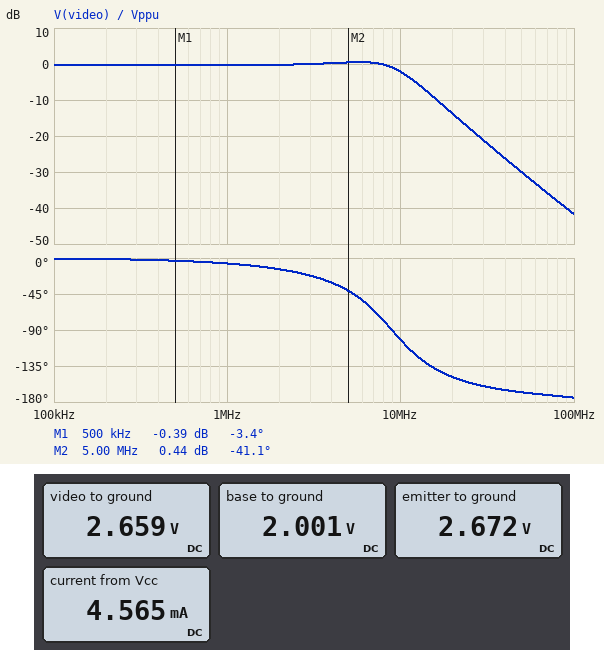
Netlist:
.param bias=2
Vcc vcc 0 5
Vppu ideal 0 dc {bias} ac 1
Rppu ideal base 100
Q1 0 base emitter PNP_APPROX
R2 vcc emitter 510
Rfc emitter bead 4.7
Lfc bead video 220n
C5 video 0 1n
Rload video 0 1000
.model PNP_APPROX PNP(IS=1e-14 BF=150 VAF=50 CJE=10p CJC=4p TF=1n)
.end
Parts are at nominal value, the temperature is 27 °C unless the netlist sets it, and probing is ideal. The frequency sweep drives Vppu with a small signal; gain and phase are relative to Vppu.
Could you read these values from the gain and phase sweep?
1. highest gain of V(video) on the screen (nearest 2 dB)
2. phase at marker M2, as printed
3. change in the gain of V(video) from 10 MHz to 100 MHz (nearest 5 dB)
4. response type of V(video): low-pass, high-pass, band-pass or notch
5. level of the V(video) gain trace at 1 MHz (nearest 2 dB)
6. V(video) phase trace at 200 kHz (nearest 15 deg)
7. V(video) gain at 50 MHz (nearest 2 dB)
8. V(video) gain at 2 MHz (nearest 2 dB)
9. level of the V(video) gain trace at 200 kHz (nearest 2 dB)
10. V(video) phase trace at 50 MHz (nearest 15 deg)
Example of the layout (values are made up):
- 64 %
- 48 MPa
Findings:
- 0 dB
- -41.1 deg
- -40 dB
- low-pass
- 0 dB
- 0 deg
- -30 dB
- 0 dB
- 0 dB
- -165 deg
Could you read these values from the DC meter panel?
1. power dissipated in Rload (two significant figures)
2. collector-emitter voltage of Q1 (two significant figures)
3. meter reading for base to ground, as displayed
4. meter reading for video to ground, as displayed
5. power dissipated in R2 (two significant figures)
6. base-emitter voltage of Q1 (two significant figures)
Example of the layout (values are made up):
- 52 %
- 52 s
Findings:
- 7.1 mW
- -2.7 V
- 2.001 V
- 2.659 V
- 11 mW
- -670 mV
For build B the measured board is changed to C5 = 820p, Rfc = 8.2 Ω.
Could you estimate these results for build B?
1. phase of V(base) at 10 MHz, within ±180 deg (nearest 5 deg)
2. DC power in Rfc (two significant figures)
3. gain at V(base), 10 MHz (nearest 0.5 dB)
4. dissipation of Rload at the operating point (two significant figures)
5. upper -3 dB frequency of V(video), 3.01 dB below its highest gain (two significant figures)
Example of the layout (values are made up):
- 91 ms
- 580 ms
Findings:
- -20 deg
- 58 µW
- 0 dB
- 7.0 mW
- 11 MHz
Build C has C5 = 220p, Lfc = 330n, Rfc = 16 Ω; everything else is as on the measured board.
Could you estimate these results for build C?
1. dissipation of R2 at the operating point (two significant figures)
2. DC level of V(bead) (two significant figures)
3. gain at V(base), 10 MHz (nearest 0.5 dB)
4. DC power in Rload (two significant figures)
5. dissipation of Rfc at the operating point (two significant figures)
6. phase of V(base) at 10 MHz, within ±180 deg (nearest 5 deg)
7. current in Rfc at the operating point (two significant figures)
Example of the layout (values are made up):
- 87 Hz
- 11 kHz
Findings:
- 11 mW
- 2.6 V
- 0.5 dB
- 6.9 mW
- 110 µW
- -5 deg
- 2.6 mA
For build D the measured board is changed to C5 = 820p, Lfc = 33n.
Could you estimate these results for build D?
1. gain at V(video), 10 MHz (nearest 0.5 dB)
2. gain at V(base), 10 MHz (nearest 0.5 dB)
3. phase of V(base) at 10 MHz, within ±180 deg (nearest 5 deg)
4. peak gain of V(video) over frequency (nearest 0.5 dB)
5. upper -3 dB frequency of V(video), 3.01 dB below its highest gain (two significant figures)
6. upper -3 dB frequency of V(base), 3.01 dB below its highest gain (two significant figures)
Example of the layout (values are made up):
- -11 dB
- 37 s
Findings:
- -1.5 dB
- 1.0 dB
- -15 deg
- -0.5 dB
- 14 MHz
- 22 MHz
